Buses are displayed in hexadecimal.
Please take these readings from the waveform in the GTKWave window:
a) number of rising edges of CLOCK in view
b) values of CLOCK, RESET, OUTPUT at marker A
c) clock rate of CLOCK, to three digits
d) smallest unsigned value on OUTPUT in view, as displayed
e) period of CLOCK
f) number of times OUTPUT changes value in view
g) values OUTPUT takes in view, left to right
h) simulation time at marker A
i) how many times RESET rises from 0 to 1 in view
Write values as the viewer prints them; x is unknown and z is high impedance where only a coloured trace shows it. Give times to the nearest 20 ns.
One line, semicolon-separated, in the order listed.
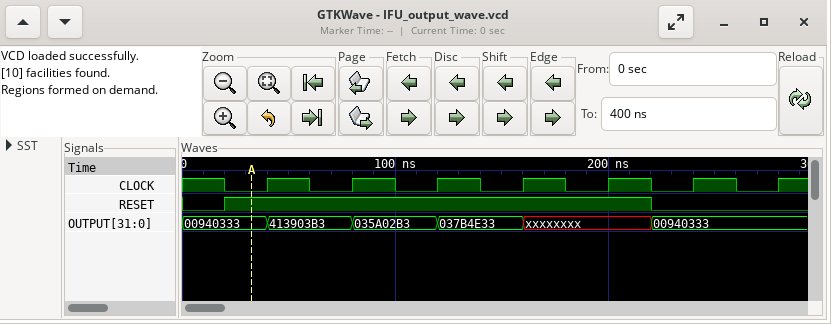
7; CLOCK=0, RESET=1, OUTPUT=00940333; 25.0 MHz; 00940333; 40 ns; 5; 00940333, 413903B3, 035A02B3, 037B4E33, xxxxxxxx, 00940333; 40 ns; 1
